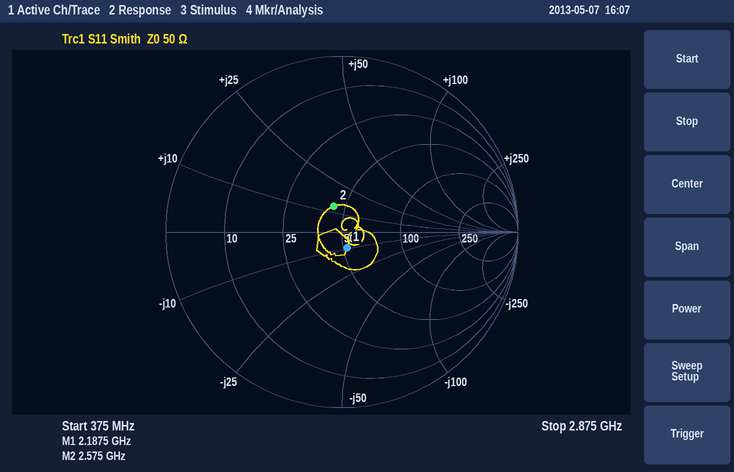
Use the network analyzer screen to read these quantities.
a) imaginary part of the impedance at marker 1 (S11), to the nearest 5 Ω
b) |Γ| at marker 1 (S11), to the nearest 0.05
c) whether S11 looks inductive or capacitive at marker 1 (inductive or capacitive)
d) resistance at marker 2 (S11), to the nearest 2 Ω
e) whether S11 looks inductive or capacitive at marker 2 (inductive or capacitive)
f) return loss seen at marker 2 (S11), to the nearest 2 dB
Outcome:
-10 Ω
0.10
capacitive
44 Ω
inductive
16 dB
